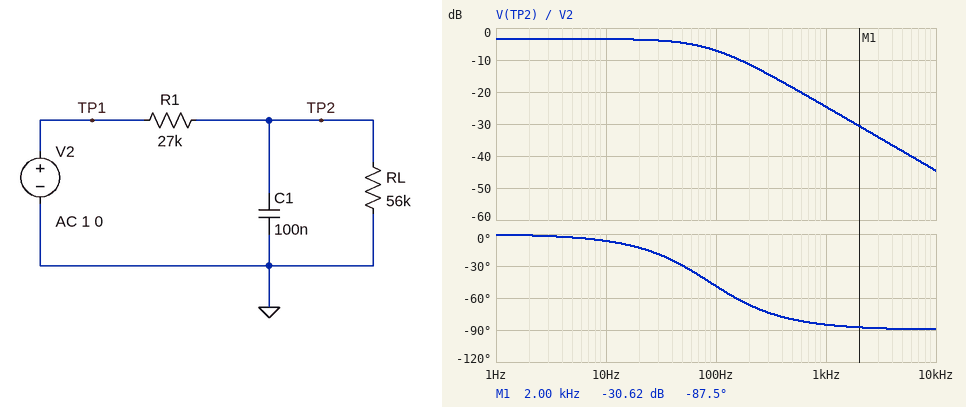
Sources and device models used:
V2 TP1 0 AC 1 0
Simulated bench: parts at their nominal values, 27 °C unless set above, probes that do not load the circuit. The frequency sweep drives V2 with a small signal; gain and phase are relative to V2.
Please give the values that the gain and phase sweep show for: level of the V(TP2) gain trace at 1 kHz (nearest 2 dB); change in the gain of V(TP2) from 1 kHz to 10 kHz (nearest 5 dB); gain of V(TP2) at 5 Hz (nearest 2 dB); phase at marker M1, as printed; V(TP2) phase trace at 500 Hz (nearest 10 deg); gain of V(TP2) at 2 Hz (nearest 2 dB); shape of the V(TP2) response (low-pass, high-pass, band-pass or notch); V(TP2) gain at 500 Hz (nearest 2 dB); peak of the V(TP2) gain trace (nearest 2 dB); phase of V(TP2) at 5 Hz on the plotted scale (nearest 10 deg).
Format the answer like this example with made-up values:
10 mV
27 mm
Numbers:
-24 dB
-20 dB
-4 dB
-87.5 deg
-80 deg
-4 dB
low-pass
-18 dB
-4 dB
0 deg
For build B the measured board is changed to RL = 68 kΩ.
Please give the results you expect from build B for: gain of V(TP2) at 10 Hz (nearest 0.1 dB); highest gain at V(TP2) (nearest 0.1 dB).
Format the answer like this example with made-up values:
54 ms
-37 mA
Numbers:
-3.0 dB
-2.9 dB
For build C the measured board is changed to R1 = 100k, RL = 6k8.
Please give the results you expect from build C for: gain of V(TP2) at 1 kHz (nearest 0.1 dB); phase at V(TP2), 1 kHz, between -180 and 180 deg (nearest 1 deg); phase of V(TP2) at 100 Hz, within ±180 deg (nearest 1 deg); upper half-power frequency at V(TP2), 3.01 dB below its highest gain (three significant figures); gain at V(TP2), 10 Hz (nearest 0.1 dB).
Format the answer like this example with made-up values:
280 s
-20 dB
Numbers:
-36.2 dB
-76 deg
-22 deg
250 Hz
-23.9 dB
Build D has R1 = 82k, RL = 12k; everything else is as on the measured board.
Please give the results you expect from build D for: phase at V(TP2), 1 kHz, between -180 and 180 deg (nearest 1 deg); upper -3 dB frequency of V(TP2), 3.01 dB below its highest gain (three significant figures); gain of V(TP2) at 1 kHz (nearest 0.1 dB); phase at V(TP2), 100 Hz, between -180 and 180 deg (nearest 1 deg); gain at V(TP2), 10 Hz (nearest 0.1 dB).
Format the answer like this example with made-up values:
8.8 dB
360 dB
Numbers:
-81 deg
152 Hz
-34.3 dB
-33 deg
-17.9 dB
